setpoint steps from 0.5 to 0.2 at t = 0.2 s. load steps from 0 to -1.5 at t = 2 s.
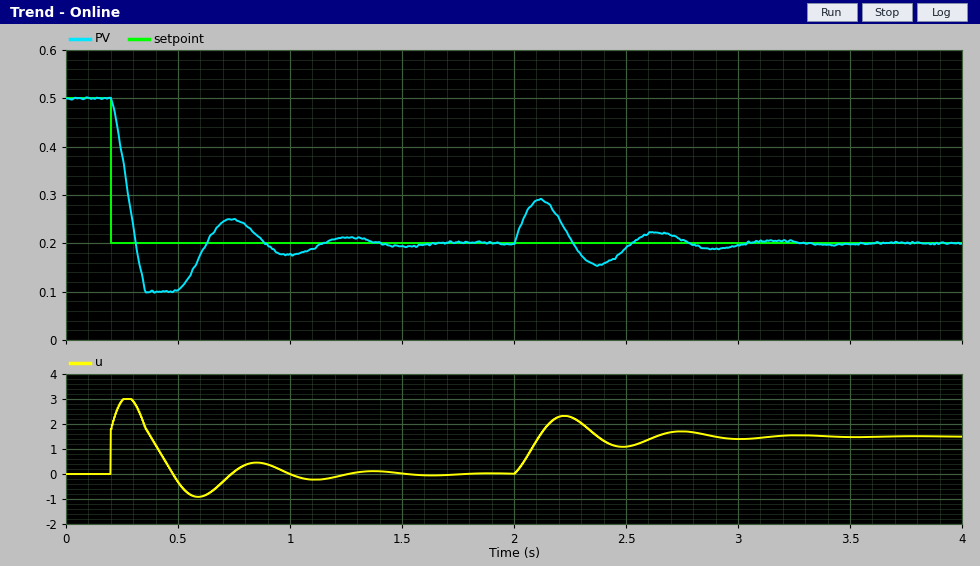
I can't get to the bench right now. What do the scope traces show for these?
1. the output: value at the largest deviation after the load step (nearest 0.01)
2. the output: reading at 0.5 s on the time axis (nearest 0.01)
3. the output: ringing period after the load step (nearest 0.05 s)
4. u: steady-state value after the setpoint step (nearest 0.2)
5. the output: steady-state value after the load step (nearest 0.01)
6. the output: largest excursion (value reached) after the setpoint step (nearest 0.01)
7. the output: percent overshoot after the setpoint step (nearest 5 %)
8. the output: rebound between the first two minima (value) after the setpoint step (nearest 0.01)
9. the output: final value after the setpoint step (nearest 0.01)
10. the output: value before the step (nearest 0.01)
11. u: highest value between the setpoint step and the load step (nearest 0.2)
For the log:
0.29
0.10
0.50 s
0.0
0.20
0.10
35 %
0.25
0.20
0.50
3.0
